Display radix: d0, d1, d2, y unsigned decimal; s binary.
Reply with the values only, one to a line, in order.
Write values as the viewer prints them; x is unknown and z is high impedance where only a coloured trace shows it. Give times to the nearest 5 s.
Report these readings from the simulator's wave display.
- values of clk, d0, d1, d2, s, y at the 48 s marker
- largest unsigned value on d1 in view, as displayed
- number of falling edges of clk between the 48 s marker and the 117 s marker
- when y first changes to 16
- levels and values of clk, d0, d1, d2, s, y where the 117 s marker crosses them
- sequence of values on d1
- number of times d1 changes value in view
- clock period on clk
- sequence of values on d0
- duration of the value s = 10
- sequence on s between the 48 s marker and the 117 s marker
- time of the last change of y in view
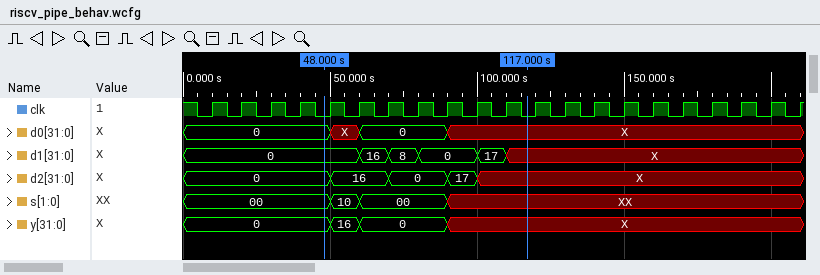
clk=0, d0=0, d1=0, d2=0, s=00, y=0
17
7
50 s
clk=0, d0=X, d1=X, d2=X, s=XX, y=X
0, 16, 8, 0, 17, X
5
10 s
0, X, 0, X
10 s
00, 10, 00, XX
90 s
